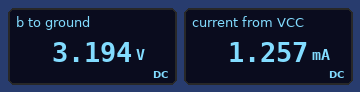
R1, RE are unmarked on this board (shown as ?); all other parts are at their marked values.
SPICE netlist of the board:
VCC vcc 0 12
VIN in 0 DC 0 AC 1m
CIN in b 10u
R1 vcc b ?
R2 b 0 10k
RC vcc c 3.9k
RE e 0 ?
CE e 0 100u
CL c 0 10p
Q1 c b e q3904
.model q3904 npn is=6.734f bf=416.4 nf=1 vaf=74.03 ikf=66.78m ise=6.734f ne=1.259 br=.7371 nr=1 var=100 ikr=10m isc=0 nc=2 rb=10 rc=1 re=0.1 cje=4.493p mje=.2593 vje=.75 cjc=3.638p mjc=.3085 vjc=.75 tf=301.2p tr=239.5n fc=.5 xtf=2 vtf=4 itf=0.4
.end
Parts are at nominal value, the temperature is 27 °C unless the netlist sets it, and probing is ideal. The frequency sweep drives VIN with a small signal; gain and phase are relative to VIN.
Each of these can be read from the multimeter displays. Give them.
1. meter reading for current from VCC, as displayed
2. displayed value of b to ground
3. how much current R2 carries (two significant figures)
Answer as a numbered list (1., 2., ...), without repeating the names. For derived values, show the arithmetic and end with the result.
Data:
1. 1.257 mA
2. 3.194 V
3. (3.194 V) / 10 kΩ = 320 µA
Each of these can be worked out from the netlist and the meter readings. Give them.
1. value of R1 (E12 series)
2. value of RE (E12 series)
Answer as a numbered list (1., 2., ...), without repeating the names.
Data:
1. 27 kΩ
2. 2.7 kΩ
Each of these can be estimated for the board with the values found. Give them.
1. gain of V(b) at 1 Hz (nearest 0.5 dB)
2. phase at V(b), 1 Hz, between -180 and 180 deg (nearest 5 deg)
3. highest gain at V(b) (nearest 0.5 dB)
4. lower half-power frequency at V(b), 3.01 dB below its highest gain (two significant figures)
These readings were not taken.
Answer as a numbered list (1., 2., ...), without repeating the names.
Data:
1. -8.0 dB
2. 65 deg
3. 0 dB
4. 2.4 Hz
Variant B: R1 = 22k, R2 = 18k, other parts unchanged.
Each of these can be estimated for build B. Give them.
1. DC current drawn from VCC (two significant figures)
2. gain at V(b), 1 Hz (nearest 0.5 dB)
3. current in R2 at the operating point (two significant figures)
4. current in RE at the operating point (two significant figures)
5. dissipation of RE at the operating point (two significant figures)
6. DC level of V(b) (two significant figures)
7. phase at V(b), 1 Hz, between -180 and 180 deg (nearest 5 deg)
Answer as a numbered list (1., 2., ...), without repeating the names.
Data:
1. 2.0 mA
2. -6.0 dB
3. 290 µA
4. 1.7 mA
5. 7.8 mW
6. 5.3 V
7. 55 deg
